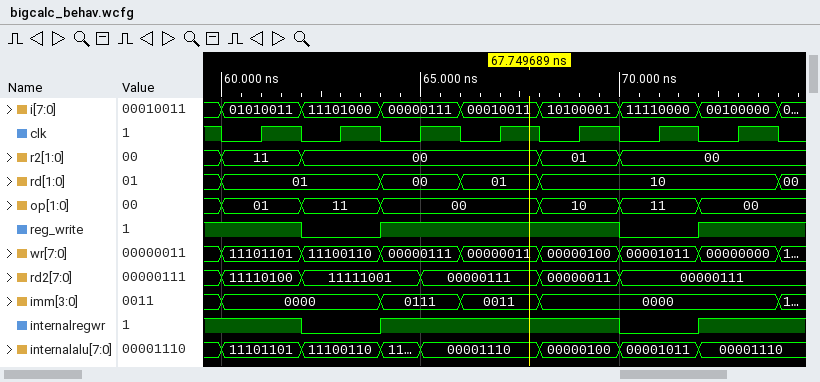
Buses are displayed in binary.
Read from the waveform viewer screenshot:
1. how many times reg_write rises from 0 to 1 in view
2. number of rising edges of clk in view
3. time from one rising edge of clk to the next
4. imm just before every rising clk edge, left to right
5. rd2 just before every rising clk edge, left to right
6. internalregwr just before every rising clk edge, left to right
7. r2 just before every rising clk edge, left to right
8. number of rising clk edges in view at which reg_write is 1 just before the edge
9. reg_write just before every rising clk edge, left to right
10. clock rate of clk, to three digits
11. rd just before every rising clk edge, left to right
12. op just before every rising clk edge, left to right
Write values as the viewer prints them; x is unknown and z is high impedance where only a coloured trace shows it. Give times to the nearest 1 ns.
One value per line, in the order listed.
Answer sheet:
2
7
2 ns
0000, 0000, 0111, 0011, 0000, 0000, 0000
11110100, 11111001, 11111001, 00000111, 00000011, 00000111, 00000111
1 0 1 1 1 0 1
11, 00, 00, 00, 01, 00, 00
5
1 0 1 1 1 0 1
500 MHz
01, 01, 00, 01, 10, 10, 10
01, 11, 00, 00, 10, 11, 00
